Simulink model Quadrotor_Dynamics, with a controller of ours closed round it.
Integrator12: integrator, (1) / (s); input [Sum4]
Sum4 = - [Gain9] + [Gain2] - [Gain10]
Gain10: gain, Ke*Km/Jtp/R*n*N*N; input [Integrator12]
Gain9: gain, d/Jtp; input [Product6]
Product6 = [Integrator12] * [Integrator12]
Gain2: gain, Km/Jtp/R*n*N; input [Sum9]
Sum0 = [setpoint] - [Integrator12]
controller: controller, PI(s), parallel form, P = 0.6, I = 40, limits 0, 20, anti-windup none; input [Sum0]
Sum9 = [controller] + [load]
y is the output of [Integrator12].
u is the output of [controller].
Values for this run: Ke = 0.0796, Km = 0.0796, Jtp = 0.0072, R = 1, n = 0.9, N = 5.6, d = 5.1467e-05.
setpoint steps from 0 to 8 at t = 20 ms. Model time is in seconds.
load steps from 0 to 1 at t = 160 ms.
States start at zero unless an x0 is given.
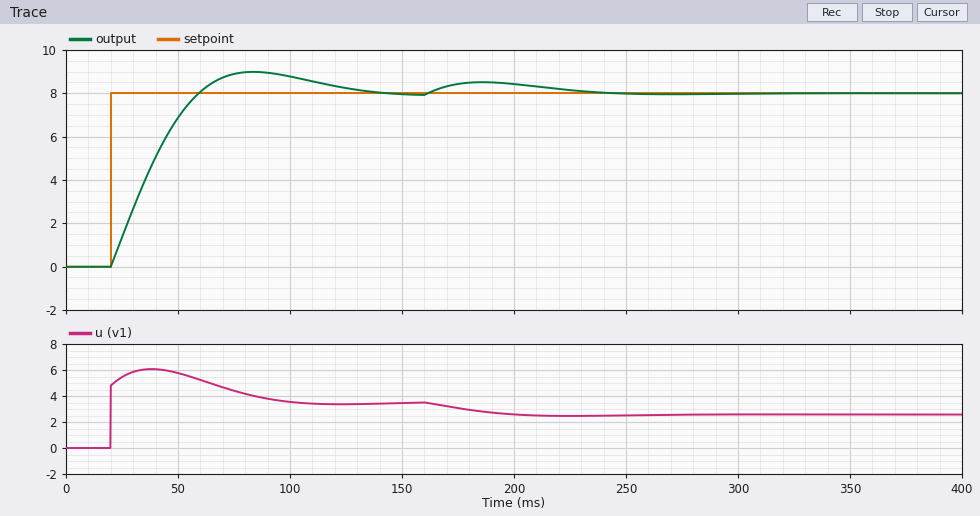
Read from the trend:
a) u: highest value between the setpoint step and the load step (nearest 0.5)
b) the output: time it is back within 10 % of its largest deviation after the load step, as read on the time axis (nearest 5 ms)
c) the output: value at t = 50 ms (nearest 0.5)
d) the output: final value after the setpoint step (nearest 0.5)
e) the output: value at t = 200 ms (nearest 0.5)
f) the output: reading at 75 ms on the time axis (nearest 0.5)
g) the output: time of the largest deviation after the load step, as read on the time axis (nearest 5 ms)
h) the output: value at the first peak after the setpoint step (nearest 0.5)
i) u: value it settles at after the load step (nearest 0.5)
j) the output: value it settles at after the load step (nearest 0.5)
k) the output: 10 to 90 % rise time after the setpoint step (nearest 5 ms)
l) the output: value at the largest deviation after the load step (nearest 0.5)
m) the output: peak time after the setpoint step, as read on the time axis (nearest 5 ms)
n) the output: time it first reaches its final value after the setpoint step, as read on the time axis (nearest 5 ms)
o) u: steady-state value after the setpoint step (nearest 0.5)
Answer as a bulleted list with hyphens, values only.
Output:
- 6.0
- 235 ms
- 7.0
- 8.0
- 8.5
- 9.0
- 185 ms
- 9.0
- 2.5
- 8.0
- 30 ms
- 8.5
- 85 ms
- 60 ms
- 3.5
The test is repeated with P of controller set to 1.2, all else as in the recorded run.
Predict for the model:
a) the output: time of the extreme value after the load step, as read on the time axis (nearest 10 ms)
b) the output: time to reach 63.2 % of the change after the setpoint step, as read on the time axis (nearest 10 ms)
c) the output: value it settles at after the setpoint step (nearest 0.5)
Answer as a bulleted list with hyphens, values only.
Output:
- 180 ms
- 30 ms
- 8.0
